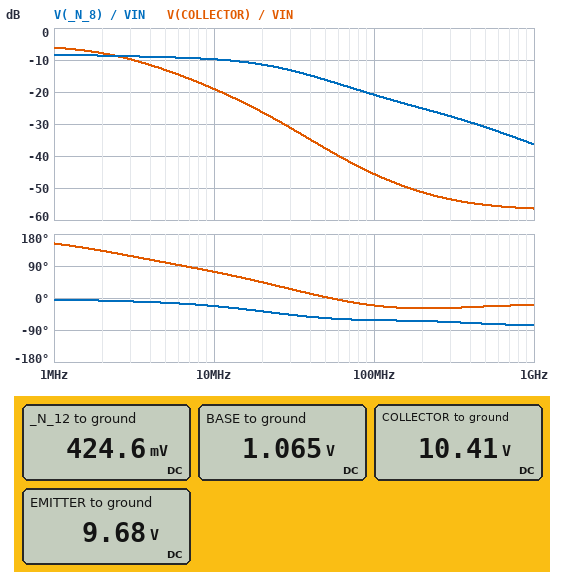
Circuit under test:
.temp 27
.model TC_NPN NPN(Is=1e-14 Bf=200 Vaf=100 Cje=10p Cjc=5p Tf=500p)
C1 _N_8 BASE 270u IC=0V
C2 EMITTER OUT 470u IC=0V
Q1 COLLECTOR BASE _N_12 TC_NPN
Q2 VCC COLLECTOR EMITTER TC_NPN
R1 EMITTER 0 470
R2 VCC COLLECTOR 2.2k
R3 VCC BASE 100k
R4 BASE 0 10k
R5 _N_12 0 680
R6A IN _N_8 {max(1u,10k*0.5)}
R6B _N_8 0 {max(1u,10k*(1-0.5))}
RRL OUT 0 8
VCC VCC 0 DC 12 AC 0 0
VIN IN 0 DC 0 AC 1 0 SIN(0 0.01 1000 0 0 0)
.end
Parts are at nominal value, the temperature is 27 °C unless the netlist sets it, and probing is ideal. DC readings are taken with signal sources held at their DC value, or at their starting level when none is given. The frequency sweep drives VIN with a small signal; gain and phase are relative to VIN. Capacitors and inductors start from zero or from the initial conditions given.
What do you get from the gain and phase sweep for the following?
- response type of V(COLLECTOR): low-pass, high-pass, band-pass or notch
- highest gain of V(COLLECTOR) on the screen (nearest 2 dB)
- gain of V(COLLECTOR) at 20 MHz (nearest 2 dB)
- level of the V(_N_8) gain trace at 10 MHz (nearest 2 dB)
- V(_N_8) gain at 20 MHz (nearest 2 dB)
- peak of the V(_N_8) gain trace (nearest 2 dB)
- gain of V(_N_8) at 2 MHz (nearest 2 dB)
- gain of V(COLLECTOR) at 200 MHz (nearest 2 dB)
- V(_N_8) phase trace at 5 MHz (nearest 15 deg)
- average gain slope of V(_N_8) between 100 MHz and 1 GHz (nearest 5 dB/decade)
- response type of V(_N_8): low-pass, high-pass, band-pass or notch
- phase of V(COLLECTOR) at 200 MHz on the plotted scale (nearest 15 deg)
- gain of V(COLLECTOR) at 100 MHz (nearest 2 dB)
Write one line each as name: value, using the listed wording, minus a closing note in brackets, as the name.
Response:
response type of V(COLLECTOR): low-pass, high-pass, band-pass or notch: low-pass
highest gain of V(COLLECTOR) on the screen: -6 dB
gain of V(COLLECTOR) at 20 MHz: -26 dB
level of the V(_N_8) gain trace at 10 MHz: -10 dB
V(_N_8) gain at 20 MHz: -12 dB
peak of the V(_N_8) gain trace: -8 dB
gain of V(_N_8) at 2 MHz: -8 dB
gain of V(COLLECTOR) at 200 MHz: -52 dB
V(_N_8) phase trace at 5 MHz: -15 deg
average gain slope of V(_N_8) between 100 MHz and 1 GHz: -15 dB/decade
response type of V(_N_8): low-pass, high-pass, band-pass or notch: low-pass
phase of V(COLLECTOR) at 200 MHz on the plotted scale: -30 deg
gain of V(COLLECTOR) at 100 MHz: -46 dB
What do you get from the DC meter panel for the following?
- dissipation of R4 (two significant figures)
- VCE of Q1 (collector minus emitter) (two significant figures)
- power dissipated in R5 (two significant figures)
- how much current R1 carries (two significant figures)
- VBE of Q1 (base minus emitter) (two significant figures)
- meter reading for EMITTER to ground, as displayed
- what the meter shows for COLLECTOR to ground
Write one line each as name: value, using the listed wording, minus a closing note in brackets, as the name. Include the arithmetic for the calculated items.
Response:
dissipation of R4: (1.065 V)^2 / 10 kΩ = 110 µW
VCE of Q1 (collector minus emitter): 10.41 V - 424.6 mV = 10 V
power dissipated in R5: (424.6 mV)^2 / 680 Ω = 270 µW
how much current R1 carries: (9.68 V) / 470 Ω = 21 mA
VBE of Q1 (base minus emitter): 1.065 V - 424.6 mV = 640 mV
meter reading for EMITTER to ground, as displayed: 9.68 V
what the meter shows for COLLECTOR to ground: 10.41 V
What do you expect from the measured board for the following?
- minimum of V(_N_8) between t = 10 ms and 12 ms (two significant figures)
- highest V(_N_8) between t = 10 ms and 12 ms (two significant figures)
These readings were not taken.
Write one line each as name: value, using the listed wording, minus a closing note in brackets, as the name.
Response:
minimum of V(_N_8) between t = 10 ms and 12 ms: 230 mV
highest V(_N_8) between t = 10 ms and 12 ms: 240 mV
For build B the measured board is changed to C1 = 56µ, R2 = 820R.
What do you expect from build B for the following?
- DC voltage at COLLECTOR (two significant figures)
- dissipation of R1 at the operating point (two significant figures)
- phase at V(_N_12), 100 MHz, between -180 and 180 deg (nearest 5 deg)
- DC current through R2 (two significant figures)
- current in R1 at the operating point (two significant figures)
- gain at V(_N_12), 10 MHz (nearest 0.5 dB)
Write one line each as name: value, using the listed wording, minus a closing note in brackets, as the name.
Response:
DC voltage at COLLECTOR: 11 V
dissipation of R1 at the operating point: 240 mW
phase at V(_N_12), 100 MHz, between -180 and 180 deg: -60 deg
DC current through R2: 730 µA
current in R1 at the operating point: 23 mA
gain at V(_N_12), 10 MHz: -10.0 dB
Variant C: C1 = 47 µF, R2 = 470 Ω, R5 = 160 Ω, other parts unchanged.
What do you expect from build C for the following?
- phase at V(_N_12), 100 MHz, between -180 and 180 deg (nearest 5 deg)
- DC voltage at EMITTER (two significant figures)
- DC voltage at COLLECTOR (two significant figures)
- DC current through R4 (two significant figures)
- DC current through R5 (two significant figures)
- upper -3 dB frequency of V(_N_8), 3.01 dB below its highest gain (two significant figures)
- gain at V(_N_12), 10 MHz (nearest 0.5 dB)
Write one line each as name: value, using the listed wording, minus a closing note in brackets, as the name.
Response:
phase at V(_N_12), 100 MHz, between -180 and 180 deg: -65 deg
DC voltage at EMITTER: 10 V
DC voltage at COLLECTOR: 11 V
DC current through R4: 100 µA
DC current through R5: 2.1 mA
upper -3 dB frequency of V(_N_8), 3.01 dB below its highest gain: 7.7 MHz
gain at V(_N_12), 10 MHz: -13.0 dB
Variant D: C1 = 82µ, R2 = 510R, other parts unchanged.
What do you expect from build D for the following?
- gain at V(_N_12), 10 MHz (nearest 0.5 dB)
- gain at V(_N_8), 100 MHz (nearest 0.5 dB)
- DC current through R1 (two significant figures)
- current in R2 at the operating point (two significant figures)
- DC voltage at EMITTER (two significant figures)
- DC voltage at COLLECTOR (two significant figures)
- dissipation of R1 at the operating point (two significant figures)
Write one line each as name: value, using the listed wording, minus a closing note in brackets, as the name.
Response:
gain at V(_N_12), 10 MHz: -10.0 dB
gain at V(_N_8), 100 MHz: -20.5 dB
DC current through R1: 23 mA
current in R2 at the operating point: 740 µA
DC voltage at EMITTER: 11 V
DC voltage at COLLECTOR: 12 V
dissipation of R1 at the operating point: 250 mW
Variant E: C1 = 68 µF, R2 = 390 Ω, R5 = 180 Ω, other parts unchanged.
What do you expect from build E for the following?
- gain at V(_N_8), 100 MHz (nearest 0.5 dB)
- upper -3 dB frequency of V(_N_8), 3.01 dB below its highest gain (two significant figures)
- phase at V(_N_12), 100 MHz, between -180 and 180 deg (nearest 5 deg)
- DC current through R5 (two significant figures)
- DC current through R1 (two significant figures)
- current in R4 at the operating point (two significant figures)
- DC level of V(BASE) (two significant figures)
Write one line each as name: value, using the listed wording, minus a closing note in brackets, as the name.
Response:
gain at V(_N_8), 100 MHz: -25.0 dB
upper -3 dB frequency of V(_N_8), 3.01 dB below its highest gain: 9.0 MHz
phase at V(_N_12), 100 MHz, between -180 and 180 deg: -65 deg
DC current through R5: 1.9 mA
DC current through R1: 22 mA
current in R4 at the operating point: 100 µA
DC level of V(BASE): 1.0 V
